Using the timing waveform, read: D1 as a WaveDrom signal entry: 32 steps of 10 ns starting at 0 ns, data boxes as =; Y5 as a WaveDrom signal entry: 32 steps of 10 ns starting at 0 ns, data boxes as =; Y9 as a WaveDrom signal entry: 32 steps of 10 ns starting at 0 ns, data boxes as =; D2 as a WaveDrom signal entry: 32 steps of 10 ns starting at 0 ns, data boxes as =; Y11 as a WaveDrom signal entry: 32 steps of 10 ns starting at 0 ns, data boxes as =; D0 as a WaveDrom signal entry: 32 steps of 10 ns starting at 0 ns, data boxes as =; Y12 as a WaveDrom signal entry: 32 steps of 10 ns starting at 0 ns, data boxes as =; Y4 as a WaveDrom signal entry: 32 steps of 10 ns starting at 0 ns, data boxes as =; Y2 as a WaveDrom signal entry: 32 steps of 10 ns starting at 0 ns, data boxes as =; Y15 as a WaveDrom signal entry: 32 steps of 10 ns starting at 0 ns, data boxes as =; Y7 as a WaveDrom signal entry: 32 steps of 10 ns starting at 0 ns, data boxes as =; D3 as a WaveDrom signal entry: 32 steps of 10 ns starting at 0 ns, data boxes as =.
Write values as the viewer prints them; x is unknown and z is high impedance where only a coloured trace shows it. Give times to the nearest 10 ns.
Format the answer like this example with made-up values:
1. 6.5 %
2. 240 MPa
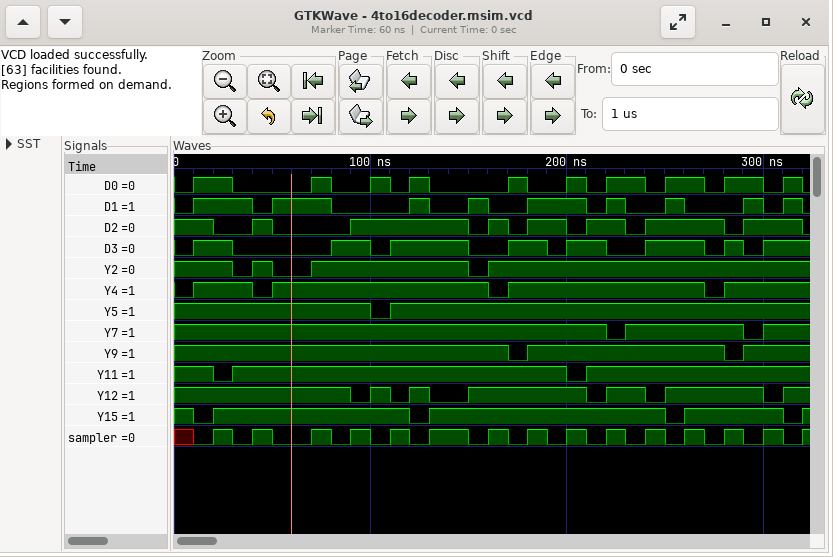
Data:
1. {name: 'D1', wave: '01..01..0...10.10.1..010.10..101'}
2. {name: 'Y5', wave: '1.........01....................'}
3. {name: 'Y9', wave: '1................01.........01..'}
4. {name: 'D2', wave: '1.0.10...1.....0101.01.01...01..'}
5. {name: 'Y11', wave: '1.01................01..........'}
6. {name: 'D0', wave: '01.0...10.1010...10.101.01.01.01'}
7. {name: 'Y12', wave: '1........01010.1.....01.01....01'}
8. {name: 'Y4', wave: '01..01..........01.........01...'}
9. {name: 'Y2', wave: '1..010.1.......01...............'}
10. {name: 'Y15', wave: '101.........01...........01....0'}
11. {name: 'Y7', wave: '1.....................01.....01.'}
12. {name: 'D3', wave: '01.0....1.01...0.1.01.0.1..0101.'}
